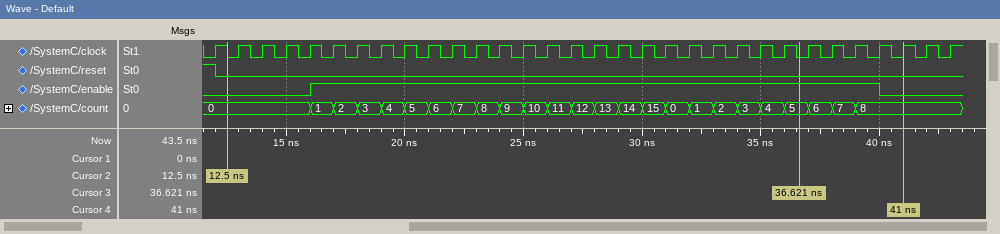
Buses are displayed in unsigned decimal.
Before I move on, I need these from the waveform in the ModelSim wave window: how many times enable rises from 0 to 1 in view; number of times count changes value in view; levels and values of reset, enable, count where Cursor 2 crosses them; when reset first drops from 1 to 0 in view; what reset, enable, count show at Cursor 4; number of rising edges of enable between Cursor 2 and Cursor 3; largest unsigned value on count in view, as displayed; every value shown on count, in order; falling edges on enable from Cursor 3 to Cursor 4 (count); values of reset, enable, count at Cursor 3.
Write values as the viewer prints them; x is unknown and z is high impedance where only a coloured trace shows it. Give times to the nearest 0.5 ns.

1
24
reset=0, enable=0, count=0
12 ns
reset=0, enable=0, count=8
1
15
0, 1, 2, 3, 4, 5, 6, 7, 8, 9, 10, 11, 12, 13, 14, 15, 0, 1, 2, 3, 4, 5, 6, 7, 8
1
reset=0, enable=1, count=5
